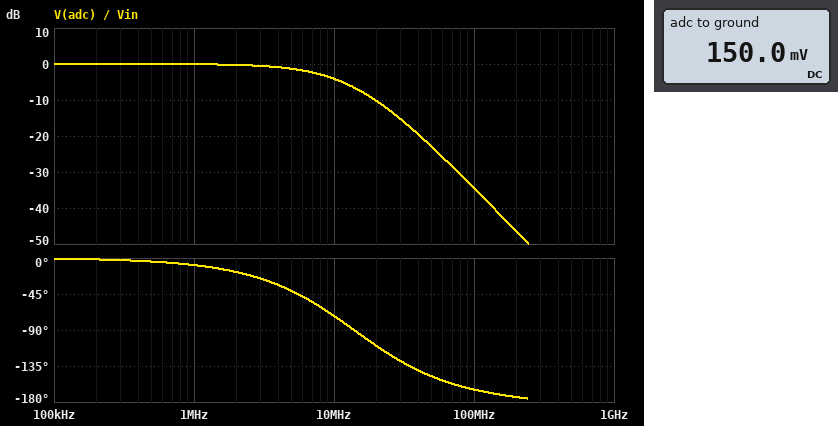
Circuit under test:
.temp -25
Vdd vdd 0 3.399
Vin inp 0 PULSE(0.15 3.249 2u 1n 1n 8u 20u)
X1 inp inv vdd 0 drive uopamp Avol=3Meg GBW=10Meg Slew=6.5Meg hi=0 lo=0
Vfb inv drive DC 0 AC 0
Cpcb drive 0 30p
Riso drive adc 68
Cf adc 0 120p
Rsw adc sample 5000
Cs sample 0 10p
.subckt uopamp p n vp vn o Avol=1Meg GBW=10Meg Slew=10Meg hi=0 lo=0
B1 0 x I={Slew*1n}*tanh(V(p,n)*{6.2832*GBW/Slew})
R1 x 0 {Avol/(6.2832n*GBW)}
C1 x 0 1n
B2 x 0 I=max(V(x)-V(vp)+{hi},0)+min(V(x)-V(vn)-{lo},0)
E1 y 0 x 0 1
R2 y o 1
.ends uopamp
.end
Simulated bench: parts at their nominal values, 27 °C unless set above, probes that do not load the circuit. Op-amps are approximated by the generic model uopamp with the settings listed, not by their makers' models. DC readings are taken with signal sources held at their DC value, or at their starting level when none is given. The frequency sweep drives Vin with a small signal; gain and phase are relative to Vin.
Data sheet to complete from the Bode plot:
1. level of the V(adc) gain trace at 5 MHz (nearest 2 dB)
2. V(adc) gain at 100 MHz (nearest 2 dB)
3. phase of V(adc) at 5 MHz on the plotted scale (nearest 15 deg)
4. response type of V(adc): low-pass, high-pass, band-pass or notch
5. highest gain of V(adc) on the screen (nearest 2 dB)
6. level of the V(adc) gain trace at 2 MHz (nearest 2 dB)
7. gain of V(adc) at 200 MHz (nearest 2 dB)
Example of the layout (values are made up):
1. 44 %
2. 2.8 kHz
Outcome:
1. -2 dB
2. -34 dB
3. -45 deg
4. low-pass
5. 0 dB
6. 0 dB
7. -46 dB
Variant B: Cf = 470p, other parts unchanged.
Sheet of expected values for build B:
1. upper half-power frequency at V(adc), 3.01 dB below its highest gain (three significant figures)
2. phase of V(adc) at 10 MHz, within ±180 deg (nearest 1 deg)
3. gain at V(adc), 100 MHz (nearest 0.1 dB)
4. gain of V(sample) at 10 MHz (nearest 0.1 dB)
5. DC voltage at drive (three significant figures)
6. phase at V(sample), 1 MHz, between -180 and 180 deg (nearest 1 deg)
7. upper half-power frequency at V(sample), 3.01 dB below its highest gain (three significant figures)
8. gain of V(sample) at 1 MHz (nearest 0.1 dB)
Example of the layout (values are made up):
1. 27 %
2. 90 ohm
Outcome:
1. 4.13 MHz
2. -109 deg
3. -46.2 dB
4. -20.4 dB
5. 150 mV
6. -35 deg
7. 2.34 MHz
8. -0.6 dB
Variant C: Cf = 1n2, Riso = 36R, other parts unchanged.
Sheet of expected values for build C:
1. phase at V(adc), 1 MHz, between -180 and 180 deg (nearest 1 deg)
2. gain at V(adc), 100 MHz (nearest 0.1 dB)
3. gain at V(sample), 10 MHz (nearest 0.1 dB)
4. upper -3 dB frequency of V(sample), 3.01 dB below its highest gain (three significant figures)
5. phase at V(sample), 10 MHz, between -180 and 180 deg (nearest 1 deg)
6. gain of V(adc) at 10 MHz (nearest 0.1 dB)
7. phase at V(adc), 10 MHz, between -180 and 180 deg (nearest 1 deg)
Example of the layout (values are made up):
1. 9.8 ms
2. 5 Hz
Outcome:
1. -21 deg
2. -48.9 dB
3. -22.7 dB
4. 2.11 MHz
5. 172 deg
6. -12.3 dB
7. -116 deg
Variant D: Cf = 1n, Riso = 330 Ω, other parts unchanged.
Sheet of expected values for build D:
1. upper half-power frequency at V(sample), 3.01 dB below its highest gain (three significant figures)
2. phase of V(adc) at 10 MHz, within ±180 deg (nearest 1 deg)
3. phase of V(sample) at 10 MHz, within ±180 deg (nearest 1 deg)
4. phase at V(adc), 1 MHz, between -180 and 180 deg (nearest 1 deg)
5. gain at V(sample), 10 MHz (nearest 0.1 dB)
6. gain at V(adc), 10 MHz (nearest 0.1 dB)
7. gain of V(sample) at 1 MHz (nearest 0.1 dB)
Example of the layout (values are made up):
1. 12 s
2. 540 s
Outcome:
1. 466 kHz
2. -132 deg
3. 155 deg
4. -70 deg
5. -39.7 dB
6. -29.4 dB
7. -7.8 dB
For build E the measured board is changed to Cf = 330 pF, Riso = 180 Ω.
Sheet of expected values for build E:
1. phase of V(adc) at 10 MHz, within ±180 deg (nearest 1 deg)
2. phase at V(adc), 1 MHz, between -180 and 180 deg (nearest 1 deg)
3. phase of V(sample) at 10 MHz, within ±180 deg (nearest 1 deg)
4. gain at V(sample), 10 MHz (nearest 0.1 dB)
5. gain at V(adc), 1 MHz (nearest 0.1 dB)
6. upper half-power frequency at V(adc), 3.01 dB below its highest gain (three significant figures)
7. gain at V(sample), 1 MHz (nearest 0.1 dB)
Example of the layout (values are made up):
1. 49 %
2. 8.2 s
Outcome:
1. -120 deg
2. -27 deg
3. 168 deg
4. -25.2 dB
5. -0.7 dB
6. 2.44 MHz
7. -1.1 dB
